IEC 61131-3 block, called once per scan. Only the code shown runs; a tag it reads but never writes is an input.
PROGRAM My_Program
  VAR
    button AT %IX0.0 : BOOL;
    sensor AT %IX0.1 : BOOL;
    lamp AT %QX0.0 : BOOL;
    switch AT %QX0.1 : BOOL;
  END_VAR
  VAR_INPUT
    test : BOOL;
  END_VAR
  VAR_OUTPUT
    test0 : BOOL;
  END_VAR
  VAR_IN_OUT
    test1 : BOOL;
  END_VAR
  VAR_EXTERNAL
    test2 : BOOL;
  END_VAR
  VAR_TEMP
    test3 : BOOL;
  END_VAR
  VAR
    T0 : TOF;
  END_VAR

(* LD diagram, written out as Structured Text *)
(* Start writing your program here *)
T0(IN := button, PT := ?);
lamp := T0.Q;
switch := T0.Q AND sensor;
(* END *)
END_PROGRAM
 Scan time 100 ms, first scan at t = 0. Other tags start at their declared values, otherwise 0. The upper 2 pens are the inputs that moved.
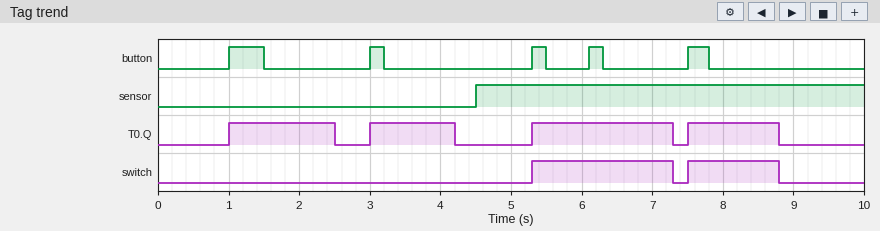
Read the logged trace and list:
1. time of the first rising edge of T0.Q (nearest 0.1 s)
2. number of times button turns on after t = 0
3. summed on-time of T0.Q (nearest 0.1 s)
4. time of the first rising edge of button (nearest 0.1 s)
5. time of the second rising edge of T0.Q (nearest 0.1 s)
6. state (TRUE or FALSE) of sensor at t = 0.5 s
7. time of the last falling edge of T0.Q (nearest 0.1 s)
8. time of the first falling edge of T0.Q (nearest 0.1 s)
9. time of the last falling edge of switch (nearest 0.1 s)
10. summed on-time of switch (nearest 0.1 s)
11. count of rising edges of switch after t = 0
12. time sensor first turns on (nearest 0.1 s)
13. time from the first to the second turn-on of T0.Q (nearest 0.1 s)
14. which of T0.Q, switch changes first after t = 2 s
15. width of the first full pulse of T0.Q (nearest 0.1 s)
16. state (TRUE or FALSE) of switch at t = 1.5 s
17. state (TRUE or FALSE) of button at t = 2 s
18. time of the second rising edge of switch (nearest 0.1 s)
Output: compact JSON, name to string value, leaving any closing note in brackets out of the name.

{"time of the first rising edge of T0.Q": "1.0 s", "number of times button turns on after t = 0": "5", "summed on-time of T0.Q": "6.0 s", "time of the first rising edge of button": "1.0 s", "time of the second rising edge of T0.Q": "3.0 s", "state (TRUE or FALSE) of sensor at t = 0.5 s": "FALSE", "time of the last falling edge of T0.Q": "8.8 s", "time of the first falling edge of T0.Q": "2.5 s", "time of the last falling edge of switch": "8.8 s", "summed on-time of switch": "3.3 s", "count of rising edges of switch after t = 0": "2", "time sensor first turns on": "4.5 s", "time from the first to the second turn-on of T0.Q": "2.0 s", "which of T0.Q, switch changes first after t = 2 s": "T0.Q", "width of the first full pulse of T0.Q": "1.5 s", "state (TRUE or FALSE) of switch at t = 1.5 s": "FALSE", "state (TRUE or FALSE) of button at t = 2 s": "FALSE", "time of the second rising edge of switch": "7.5 s"}
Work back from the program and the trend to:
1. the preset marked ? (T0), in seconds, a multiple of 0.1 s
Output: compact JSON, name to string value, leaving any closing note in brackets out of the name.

{"the preset marked ? (T0), in seconds, a multiple of 0.1 s": "1.0 s"}
